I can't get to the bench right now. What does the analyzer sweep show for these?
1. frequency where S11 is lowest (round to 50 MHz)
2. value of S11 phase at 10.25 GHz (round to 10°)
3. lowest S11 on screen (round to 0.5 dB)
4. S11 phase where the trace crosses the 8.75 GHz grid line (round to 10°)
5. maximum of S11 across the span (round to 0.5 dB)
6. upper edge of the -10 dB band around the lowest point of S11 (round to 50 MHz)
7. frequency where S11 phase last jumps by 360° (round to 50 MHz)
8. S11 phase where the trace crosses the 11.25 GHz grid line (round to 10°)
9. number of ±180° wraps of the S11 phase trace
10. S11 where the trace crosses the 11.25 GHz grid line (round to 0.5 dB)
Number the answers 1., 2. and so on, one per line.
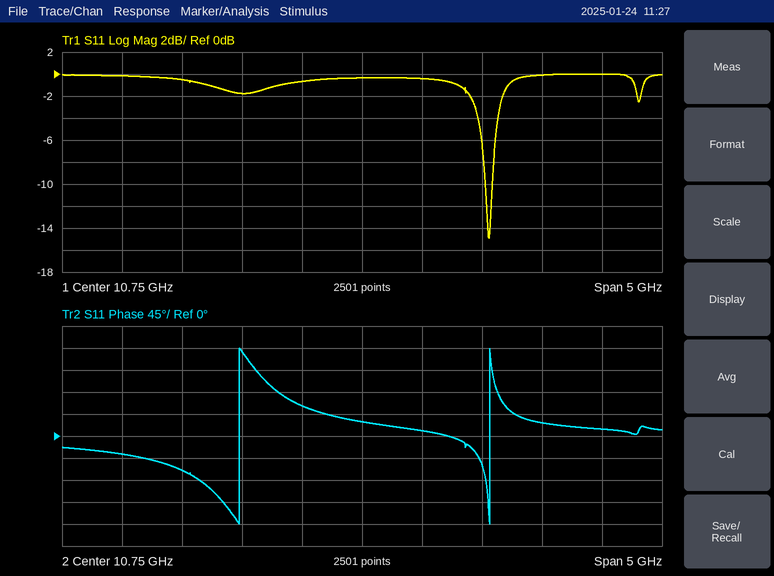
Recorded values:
1. 11.80 GHz
2. 60°
3. -15.0 dB
4. -40°
5. 0.0 dB
6. 11.85 GHz
7. 11.80 GHz
8. 10°
9. 2
10. -0.5 dB
